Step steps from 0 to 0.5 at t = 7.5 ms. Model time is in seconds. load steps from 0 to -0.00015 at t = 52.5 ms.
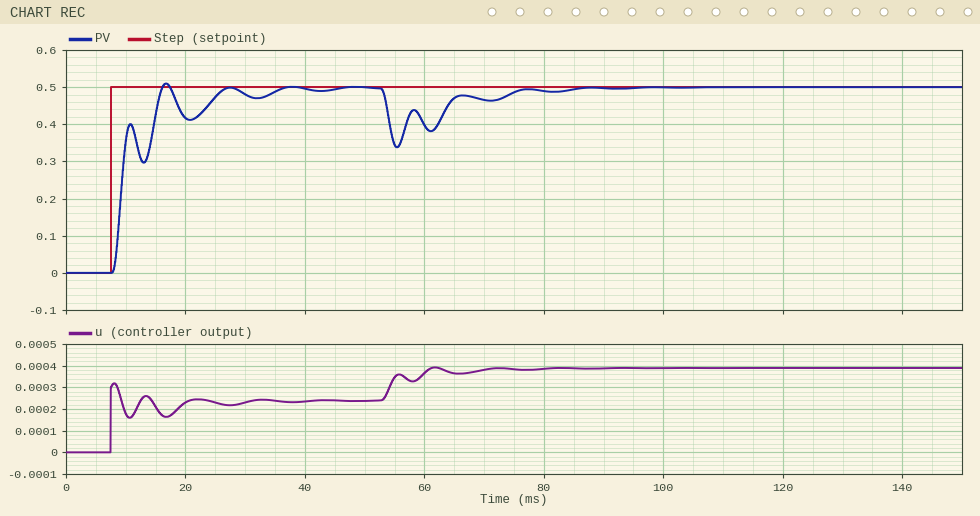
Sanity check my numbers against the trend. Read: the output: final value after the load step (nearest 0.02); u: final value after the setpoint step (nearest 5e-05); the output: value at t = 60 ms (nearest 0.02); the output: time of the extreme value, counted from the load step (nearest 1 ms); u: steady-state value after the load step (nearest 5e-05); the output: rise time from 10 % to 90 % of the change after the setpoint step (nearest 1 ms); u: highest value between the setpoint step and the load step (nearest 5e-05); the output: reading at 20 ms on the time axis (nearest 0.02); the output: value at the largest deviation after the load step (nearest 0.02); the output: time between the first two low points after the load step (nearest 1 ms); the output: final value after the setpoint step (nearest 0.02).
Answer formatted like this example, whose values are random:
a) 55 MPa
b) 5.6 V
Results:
a) 0.50
b) 0.00025
c) 0.40
d) 3 ms
e) 0.00040
f) 7 ms
g) 0.00030
h) 0.42
i) 0.34
j) 6 ms
k) 0.50
